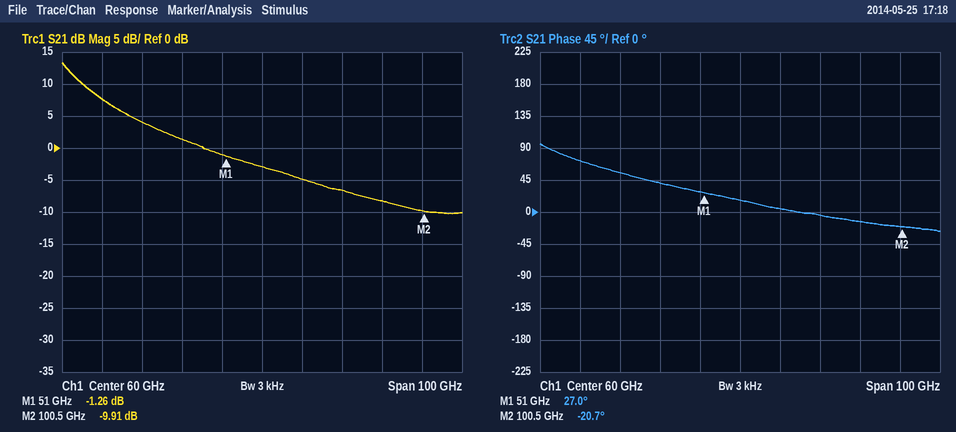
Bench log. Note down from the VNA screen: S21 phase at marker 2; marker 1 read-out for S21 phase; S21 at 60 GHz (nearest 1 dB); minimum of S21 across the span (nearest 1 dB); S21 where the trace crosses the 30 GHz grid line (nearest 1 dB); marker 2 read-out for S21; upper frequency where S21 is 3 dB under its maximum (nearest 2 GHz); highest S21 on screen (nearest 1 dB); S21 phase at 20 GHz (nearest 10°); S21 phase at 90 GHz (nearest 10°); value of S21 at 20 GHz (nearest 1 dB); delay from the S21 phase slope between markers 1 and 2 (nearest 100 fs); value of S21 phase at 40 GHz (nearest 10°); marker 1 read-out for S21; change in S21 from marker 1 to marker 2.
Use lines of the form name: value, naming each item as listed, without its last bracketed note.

S21 phase at marker 2: -20.7°
marker 1 read-out for S21 phase: 27.0°
S21 at 60 GHz: -3 dB
minimum of S21 across the span: -10 dB
S21 where the trace crosses the 30 GHz grid line: 4 dB
marker 2 read-out for S21: -9.91 dB
upper frequency where S21 is 3 dB under its maximum: 14 GHz
highest S21 on screen: 13 dB
S21 phase at 20 GHz: 70°
S21 phase at 90 GHz: -10°
value of S21 at 20 GHz: 8 dB
delay from the S21 phase slope between markers 1 and 2: 2.7 ps
value of S21 phase at 40 GHz: 40°
marker 1 read-out for S21: -1.26 dB
change in S21 from marker 1 to marker 2: -8.65 dB
